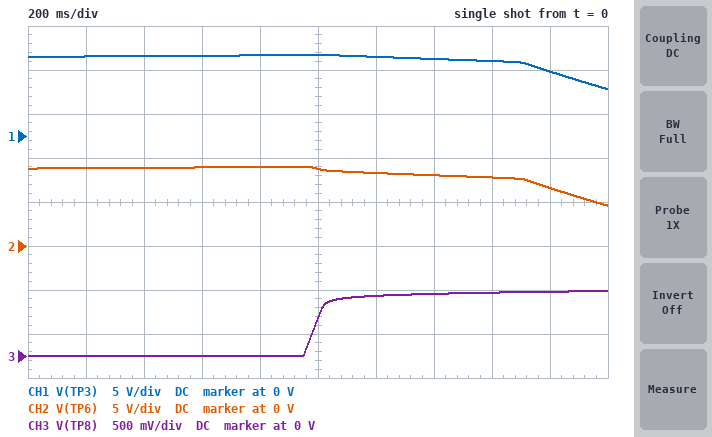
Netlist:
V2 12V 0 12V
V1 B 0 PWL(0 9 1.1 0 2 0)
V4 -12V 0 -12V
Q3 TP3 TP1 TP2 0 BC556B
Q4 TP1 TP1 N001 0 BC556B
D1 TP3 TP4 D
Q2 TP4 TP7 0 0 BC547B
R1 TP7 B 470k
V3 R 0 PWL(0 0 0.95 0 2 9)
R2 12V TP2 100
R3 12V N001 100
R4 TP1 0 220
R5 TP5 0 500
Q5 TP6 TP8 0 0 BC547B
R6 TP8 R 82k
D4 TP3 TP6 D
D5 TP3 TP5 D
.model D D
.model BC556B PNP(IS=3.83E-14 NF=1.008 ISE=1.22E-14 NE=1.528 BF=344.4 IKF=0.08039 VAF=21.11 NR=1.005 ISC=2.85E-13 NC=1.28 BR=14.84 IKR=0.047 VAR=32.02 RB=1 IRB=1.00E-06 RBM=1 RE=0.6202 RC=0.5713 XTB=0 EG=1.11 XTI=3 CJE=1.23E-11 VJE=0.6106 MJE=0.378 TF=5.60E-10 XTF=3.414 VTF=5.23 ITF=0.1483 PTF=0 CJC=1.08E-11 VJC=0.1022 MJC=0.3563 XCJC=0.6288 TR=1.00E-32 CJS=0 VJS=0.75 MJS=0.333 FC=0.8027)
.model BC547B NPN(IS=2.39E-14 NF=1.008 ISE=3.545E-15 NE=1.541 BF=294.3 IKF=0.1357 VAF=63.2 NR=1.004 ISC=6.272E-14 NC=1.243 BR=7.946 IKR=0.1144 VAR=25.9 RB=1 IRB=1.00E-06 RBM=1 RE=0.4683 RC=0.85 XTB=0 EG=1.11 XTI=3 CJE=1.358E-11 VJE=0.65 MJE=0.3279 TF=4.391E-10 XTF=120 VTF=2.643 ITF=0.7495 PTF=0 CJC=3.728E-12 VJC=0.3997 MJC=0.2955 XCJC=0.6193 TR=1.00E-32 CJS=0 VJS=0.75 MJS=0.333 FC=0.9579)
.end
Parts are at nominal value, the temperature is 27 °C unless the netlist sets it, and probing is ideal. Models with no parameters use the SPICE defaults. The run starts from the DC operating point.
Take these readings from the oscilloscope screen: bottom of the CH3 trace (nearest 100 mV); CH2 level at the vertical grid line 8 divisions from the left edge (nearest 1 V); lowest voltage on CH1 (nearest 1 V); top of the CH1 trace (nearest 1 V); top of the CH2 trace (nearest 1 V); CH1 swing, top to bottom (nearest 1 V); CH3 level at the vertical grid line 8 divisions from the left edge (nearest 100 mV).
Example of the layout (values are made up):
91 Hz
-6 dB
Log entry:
0 V
8 V
5 V
9 V
9 V
4 V
700 mV
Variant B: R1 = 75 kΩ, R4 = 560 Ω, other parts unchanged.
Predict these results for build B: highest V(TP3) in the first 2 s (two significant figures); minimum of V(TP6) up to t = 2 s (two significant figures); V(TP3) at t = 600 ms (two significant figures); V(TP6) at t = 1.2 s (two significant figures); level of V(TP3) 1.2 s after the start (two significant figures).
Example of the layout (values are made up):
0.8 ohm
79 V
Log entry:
9.1 V
140 mV
3.2 V
5.9 V
6.6 V
